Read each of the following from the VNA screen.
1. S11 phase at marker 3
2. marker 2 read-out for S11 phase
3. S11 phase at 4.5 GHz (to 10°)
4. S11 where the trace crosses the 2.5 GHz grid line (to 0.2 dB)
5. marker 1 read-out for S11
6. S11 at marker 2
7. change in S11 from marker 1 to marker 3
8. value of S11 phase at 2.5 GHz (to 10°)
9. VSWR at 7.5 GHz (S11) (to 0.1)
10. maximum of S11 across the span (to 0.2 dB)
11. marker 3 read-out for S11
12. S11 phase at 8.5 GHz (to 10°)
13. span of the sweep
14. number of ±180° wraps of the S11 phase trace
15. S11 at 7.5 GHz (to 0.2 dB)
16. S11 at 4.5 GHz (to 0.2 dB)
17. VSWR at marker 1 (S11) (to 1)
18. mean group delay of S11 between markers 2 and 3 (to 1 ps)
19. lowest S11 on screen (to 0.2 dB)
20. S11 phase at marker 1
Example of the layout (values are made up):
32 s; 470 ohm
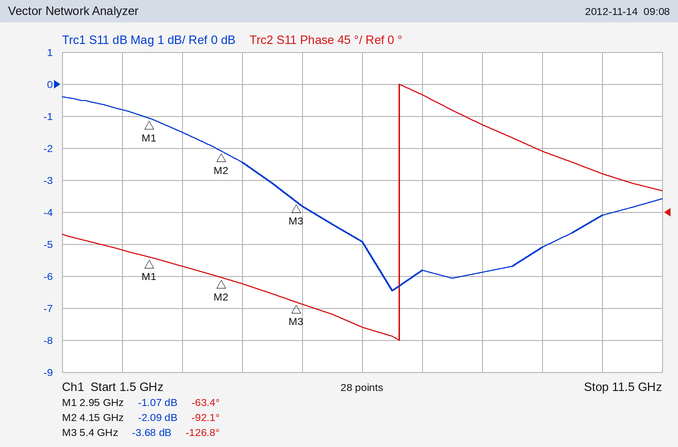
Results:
-126.8°; -92.1°; -100°; -0.8 dB; -1.07 dB; -2.09 dB; -2.61 dB; -50°; 3.1; -0.4 dB; -3.68 dB; 120°; 10 GHz; 1; -5.8 dB; -2.4 dB; 16; 77 ps; -6.4 dB; -63.4°
